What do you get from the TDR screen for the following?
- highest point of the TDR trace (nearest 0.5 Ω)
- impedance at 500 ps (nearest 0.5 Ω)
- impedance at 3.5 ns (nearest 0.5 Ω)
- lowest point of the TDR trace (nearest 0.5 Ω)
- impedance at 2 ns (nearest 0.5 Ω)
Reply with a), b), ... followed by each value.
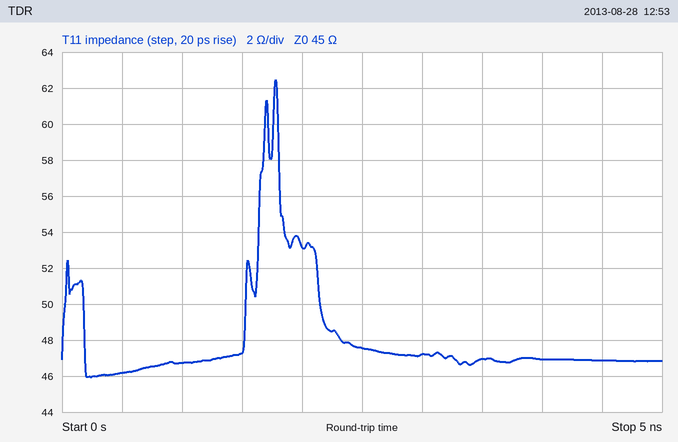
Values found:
a) 62.5 Ω
b) 46.0 Ω
c) 47.0 Ω
d) 46.0 Ω
e) 53.0 Ω
